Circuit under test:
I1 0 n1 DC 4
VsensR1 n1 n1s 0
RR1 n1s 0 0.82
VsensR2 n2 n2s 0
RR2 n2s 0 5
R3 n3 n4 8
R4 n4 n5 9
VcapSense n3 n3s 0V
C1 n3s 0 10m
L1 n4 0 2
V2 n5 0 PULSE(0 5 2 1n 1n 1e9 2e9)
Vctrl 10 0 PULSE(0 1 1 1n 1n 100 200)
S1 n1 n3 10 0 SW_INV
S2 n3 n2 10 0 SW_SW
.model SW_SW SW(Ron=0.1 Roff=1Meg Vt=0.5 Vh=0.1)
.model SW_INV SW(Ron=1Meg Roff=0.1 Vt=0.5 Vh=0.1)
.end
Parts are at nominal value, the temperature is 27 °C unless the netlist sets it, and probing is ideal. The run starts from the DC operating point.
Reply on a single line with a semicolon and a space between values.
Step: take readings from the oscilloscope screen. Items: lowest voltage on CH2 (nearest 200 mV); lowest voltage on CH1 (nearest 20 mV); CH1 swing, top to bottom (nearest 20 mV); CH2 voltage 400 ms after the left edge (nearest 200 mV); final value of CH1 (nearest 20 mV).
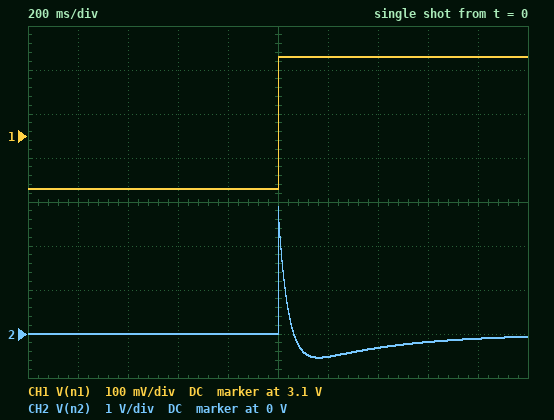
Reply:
-600 mV; 2.98 V; 300 mV; 0 V; 3.28 V
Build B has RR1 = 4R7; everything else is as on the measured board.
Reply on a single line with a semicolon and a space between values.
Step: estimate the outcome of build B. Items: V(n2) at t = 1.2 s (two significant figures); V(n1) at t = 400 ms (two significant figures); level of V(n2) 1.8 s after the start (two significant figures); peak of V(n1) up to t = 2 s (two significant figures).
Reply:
-2.1 V; 12 V; -420 mV; 19 V
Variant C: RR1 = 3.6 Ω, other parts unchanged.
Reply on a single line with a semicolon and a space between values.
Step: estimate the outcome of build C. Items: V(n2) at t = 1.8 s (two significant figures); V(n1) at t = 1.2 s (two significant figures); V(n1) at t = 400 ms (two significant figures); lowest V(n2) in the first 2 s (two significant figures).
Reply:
-350 mV; 14 V; 10 V; -1.8 V
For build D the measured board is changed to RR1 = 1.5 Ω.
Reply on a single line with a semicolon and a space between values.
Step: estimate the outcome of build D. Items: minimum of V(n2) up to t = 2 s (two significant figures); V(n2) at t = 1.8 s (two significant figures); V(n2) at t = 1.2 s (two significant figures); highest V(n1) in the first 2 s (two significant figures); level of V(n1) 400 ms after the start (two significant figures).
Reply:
-910 mV; -180 mV; -880 mV; 6.0 V; 5.1 V
